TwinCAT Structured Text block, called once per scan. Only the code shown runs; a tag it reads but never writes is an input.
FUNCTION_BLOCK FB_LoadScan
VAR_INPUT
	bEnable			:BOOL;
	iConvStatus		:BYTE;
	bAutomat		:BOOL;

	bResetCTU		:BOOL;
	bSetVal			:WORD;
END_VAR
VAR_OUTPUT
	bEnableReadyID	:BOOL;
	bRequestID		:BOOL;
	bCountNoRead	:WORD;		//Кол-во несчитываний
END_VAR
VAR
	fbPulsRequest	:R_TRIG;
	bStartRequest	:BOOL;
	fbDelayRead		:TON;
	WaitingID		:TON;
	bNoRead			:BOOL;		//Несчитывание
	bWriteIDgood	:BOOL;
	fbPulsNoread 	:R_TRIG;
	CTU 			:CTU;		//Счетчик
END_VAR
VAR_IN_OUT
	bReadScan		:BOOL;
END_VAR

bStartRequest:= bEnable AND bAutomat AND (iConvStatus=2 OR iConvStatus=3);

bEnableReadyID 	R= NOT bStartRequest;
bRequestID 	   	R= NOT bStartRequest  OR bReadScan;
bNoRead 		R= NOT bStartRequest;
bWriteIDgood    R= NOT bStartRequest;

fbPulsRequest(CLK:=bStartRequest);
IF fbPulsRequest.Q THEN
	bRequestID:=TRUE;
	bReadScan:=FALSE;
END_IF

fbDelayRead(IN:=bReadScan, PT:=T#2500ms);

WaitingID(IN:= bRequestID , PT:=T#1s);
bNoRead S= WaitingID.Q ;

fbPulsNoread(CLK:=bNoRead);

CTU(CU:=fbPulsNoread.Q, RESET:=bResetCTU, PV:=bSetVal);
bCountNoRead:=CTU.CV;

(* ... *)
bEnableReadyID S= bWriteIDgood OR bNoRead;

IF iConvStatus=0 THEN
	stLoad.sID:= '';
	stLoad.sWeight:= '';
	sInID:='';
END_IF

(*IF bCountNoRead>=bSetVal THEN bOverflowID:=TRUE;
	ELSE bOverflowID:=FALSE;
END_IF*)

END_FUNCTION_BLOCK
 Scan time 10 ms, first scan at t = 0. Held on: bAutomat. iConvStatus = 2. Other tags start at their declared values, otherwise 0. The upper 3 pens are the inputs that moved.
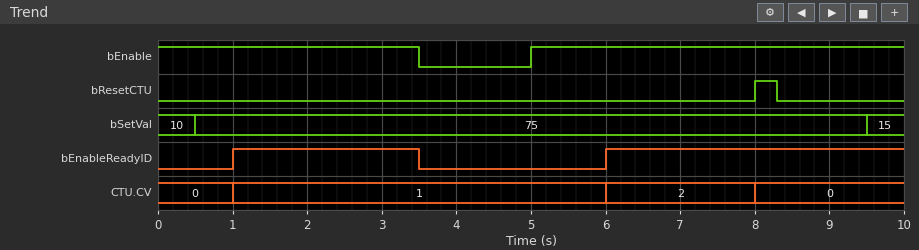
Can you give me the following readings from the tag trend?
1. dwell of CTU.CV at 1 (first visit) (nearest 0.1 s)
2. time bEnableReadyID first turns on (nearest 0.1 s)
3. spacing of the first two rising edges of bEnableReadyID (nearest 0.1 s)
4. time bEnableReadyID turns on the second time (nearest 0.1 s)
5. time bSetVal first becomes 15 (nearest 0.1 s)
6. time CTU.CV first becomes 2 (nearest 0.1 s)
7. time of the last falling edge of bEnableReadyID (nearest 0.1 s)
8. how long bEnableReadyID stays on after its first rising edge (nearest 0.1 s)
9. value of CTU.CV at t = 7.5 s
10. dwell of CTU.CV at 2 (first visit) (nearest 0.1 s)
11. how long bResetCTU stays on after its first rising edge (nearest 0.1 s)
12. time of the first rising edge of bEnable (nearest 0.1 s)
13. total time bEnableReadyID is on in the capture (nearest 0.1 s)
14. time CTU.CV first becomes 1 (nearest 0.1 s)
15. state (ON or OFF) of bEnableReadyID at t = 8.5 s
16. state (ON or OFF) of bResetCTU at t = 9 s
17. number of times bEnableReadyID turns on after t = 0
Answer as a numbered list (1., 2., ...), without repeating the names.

1. 5.0 s
2. 1.0 s
3. 5.0 s
4. 6.0 s
5. 9.5 s
6. 6.0 s
7. 3.5 s
8. 2.5 s
9. 2
10. 2.0 s
11. 0.3 s
12. 5.0 s
13. 6.5 s
14. 1.0 s
15. ON
16. OFF
17. 2
